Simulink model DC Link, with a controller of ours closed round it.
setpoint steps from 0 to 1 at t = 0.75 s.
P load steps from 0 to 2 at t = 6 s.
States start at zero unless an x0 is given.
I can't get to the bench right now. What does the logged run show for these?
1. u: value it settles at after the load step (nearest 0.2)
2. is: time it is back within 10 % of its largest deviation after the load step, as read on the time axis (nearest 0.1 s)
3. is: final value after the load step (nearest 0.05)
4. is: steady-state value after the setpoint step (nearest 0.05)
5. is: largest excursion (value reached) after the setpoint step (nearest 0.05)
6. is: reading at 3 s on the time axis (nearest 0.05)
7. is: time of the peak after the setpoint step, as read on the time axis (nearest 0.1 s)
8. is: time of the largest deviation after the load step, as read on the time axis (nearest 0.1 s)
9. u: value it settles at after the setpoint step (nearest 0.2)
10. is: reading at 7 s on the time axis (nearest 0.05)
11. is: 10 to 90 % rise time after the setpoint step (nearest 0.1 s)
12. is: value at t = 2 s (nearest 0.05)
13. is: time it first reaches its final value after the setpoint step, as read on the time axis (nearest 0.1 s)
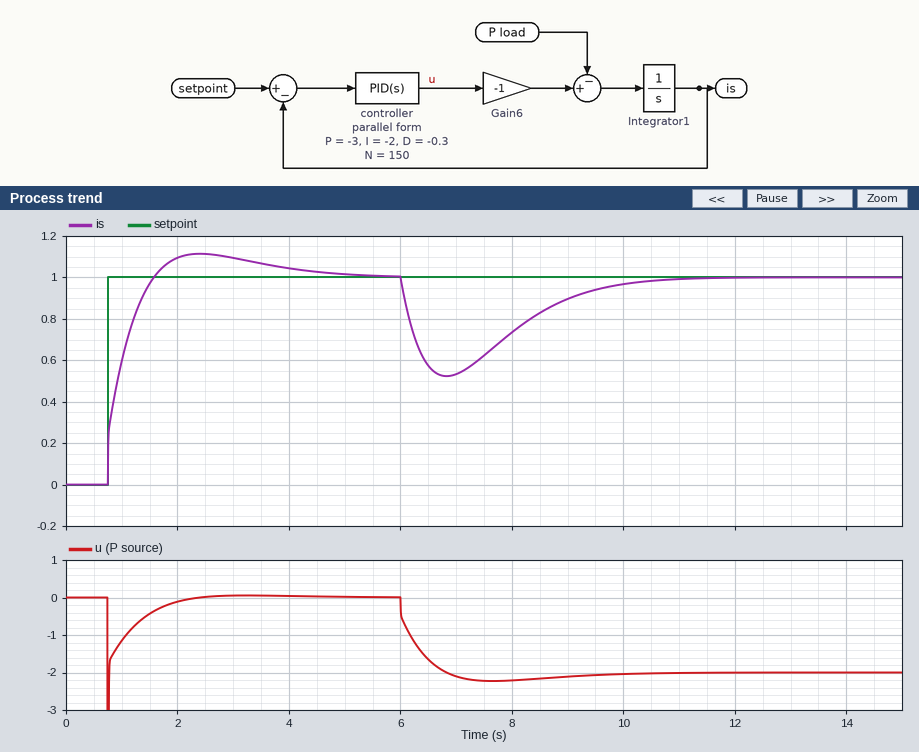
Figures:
-2.0
9.7 s
1.00
1.00
1.10
1.10
2.4 s
6.8 s
0.0
0.55
0.6 s
1.10
1.6 s
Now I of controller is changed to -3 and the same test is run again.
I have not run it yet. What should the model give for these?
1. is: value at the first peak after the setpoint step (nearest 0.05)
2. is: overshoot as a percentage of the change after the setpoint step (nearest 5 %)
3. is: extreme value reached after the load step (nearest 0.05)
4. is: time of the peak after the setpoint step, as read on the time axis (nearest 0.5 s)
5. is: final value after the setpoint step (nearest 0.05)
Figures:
1.15
15 %
0.55
2.0 s
1.00
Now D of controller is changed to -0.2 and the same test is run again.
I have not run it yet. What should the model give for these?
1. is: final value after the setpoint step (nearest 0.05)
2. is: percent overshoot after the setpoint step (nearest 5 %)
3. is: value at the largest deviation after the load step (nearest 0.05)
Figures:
1.00
10 %
0.50
